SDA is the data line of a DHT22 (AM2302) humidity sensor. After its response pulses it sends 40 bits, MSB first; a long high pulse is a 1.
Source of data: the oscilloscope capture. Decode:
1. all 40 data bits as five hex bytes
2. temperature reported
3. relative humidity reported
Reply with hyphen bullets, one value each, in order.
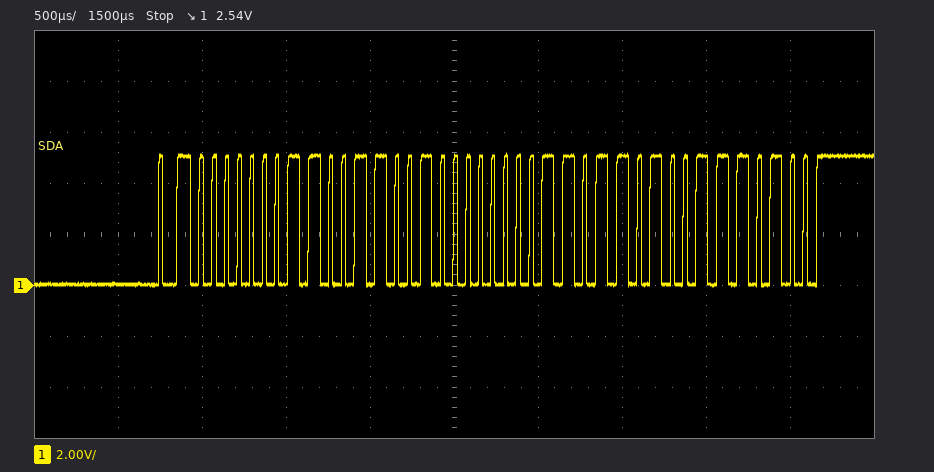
- 01 99 00 DA 74
- 21.8 °C
- 40.9 %
